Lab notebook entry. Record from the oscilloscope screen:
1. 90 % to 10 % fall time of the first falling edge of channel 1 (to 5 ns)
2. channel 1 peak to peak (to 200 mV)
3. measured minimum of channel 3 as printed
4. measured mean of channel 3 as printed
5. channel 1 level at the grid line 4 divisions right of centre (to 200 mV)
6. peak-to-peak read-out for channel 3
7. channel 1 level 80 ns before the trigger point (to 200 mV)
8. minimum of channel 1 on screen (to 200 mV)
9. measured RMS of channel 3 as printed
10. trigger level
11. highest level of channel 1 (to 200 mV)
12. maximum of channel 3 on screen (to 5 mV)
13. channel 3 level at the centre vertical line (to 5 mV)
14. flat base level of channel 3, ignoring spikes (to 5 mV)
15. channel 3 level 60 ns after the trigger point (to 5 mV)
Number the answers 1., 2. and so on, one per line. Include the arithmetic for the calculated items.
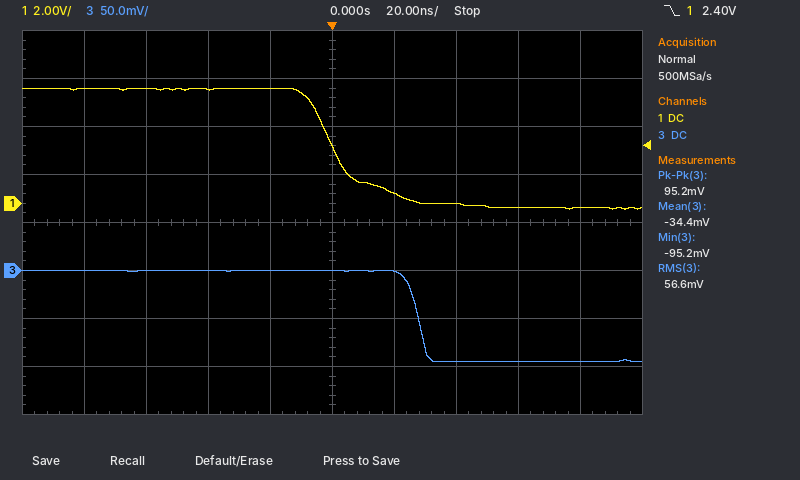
1. 30 ns
2. 4.8 V − (-200 mV) = 5.0 V
3. -95.2 mV
4. -34.4 mV
5. -200 mV
6. 95.2 mV
7. 4.8 V
8. -200 mV
9. 56.6 mV
10. 2.40 V
11. 4.8 V
12. 0 mV
13. 0 mV
14. -95 mV
15. -95 mV
